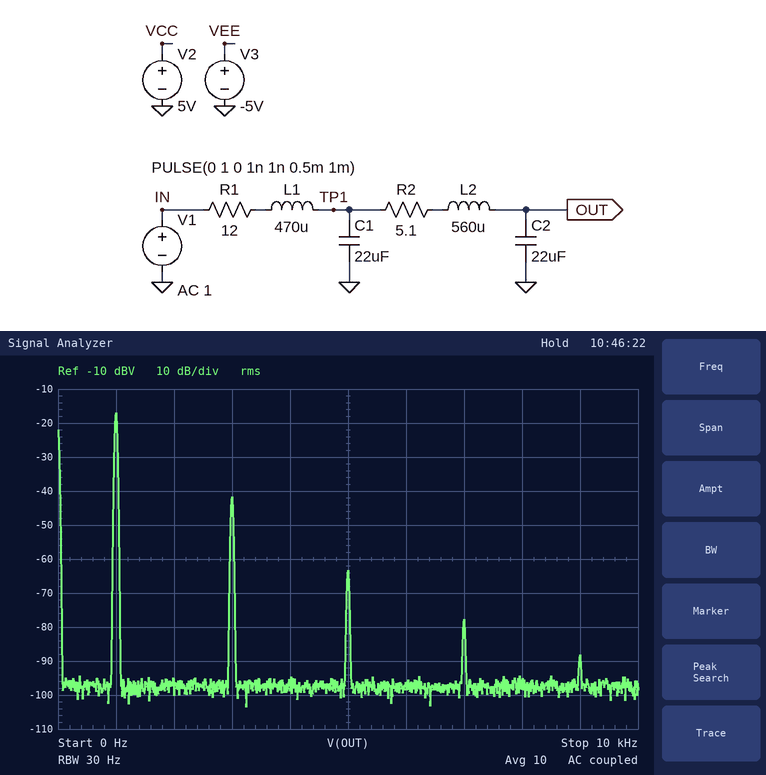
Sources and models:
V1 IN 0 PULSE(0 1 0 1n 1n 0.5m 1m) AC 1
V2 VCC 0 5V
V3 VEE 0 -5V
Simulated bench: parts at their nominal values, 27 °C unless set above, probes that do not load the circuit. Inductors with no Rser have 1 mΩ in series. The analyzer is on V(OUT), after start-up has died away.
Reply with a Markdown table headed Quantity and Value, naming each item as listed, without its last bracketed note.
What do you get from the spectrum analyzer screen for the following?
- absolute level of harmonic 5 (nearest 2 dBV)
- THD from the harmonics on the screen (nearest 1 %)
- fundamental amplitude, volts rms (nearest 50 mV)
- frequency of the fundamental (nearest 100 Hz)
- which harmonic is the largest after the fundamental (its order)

| Quantity | Value |
|---|---|
| absolute level of harmonic 5 | -64 dBV |
| THD from the harmonics on the screen | 6 % |
| fundamental amplitude, volts rms | 150 mV |
| frequency of the fundamental | 1.0 kHz |
| which harmonic is the largest after the fundamental | 3 |
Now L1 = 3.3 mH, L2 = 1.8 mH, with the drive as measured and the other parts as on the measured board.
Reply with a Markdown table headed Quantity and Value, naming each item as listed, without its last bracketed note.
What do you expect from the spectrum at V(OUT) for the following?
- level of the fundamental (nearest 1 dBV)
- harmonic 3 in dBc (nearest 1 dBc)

| Quantity | Value |
|---|---|
| level of the fundamental | -17 dBV |
| harmonic 3 in dBc | -50 dBc |
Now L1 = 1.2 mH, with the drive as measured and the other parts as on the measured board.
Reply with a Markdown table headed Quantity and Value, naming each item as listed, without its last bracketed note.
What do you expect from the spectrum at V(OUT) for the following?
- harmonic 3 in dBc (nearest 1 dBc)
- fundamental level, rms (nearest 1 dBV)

| Quantity | Value |
|---|---|
| harmonic 3 in dBc | -29 dBc |
| fundamental level, rms | -17 dBV |
